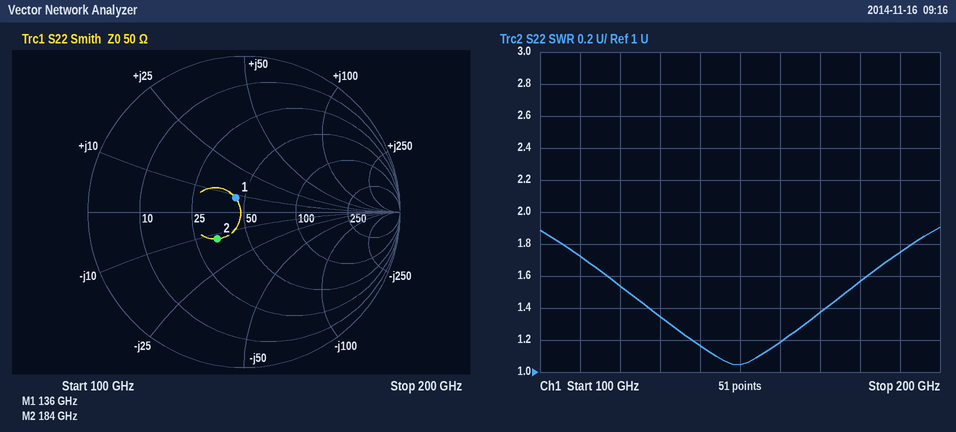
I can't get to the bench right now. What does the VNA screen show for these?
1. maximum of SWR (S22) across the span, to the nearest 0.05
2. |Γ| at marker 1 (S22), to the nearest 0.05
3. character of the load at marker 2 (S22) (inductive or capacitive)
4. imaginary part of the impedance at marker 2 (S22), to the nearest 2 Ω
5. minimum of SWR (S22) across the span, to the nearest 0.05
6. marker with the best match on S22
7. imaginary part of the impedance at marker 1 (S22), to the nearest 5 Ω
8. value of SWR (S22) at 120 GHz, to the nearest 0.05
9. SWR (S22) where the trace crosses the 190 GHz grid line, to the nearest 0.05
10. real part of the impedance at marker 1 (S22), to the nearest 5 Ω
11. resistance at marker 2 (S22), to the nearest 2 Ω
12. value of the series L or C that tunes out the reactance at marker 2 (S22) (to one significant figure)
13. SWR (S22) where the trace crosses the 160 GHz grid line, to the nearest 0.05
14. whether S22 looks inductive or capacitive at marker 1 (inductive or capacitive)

1.90
0.10
capacitive
-12 Ω
1.05
marker 1
+10 Ω
1.55
1.75
45 Ω
34 Ω
10 pH
1.20
inductive
